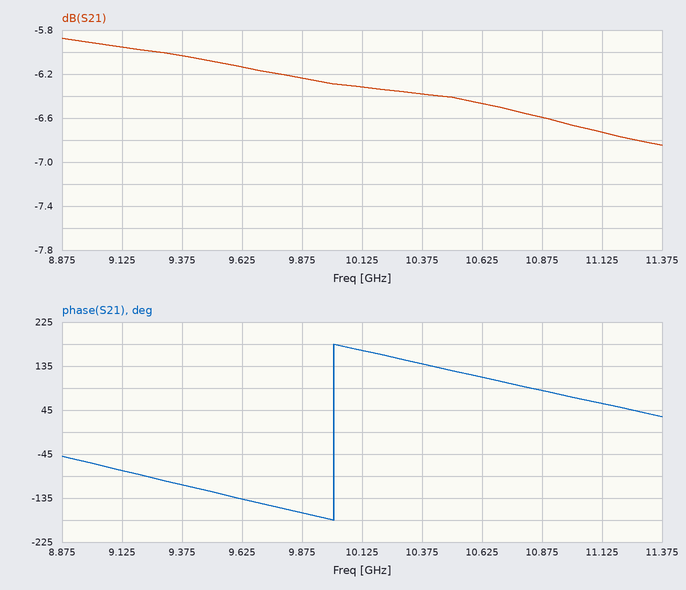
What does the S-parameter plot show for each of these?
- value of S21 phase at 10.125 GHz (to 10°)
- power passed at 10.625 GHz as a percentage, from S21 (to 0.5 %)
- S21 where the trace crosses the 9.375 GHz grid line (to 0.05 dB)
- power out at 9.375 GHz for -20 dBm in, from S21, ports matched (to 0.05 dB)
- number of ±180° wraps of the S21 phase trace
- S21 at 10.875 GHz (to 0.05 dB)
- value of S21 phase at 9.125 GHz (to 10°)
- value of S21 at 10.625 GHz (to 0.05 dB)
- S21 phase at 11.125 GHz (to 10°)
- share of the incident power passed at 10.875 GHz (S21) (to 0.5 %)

170°
22.5 %
-6.05 dB
-26.05 dBm
1
-6.60 dB
-80°
-6.45 dB
60°
22.0 %
